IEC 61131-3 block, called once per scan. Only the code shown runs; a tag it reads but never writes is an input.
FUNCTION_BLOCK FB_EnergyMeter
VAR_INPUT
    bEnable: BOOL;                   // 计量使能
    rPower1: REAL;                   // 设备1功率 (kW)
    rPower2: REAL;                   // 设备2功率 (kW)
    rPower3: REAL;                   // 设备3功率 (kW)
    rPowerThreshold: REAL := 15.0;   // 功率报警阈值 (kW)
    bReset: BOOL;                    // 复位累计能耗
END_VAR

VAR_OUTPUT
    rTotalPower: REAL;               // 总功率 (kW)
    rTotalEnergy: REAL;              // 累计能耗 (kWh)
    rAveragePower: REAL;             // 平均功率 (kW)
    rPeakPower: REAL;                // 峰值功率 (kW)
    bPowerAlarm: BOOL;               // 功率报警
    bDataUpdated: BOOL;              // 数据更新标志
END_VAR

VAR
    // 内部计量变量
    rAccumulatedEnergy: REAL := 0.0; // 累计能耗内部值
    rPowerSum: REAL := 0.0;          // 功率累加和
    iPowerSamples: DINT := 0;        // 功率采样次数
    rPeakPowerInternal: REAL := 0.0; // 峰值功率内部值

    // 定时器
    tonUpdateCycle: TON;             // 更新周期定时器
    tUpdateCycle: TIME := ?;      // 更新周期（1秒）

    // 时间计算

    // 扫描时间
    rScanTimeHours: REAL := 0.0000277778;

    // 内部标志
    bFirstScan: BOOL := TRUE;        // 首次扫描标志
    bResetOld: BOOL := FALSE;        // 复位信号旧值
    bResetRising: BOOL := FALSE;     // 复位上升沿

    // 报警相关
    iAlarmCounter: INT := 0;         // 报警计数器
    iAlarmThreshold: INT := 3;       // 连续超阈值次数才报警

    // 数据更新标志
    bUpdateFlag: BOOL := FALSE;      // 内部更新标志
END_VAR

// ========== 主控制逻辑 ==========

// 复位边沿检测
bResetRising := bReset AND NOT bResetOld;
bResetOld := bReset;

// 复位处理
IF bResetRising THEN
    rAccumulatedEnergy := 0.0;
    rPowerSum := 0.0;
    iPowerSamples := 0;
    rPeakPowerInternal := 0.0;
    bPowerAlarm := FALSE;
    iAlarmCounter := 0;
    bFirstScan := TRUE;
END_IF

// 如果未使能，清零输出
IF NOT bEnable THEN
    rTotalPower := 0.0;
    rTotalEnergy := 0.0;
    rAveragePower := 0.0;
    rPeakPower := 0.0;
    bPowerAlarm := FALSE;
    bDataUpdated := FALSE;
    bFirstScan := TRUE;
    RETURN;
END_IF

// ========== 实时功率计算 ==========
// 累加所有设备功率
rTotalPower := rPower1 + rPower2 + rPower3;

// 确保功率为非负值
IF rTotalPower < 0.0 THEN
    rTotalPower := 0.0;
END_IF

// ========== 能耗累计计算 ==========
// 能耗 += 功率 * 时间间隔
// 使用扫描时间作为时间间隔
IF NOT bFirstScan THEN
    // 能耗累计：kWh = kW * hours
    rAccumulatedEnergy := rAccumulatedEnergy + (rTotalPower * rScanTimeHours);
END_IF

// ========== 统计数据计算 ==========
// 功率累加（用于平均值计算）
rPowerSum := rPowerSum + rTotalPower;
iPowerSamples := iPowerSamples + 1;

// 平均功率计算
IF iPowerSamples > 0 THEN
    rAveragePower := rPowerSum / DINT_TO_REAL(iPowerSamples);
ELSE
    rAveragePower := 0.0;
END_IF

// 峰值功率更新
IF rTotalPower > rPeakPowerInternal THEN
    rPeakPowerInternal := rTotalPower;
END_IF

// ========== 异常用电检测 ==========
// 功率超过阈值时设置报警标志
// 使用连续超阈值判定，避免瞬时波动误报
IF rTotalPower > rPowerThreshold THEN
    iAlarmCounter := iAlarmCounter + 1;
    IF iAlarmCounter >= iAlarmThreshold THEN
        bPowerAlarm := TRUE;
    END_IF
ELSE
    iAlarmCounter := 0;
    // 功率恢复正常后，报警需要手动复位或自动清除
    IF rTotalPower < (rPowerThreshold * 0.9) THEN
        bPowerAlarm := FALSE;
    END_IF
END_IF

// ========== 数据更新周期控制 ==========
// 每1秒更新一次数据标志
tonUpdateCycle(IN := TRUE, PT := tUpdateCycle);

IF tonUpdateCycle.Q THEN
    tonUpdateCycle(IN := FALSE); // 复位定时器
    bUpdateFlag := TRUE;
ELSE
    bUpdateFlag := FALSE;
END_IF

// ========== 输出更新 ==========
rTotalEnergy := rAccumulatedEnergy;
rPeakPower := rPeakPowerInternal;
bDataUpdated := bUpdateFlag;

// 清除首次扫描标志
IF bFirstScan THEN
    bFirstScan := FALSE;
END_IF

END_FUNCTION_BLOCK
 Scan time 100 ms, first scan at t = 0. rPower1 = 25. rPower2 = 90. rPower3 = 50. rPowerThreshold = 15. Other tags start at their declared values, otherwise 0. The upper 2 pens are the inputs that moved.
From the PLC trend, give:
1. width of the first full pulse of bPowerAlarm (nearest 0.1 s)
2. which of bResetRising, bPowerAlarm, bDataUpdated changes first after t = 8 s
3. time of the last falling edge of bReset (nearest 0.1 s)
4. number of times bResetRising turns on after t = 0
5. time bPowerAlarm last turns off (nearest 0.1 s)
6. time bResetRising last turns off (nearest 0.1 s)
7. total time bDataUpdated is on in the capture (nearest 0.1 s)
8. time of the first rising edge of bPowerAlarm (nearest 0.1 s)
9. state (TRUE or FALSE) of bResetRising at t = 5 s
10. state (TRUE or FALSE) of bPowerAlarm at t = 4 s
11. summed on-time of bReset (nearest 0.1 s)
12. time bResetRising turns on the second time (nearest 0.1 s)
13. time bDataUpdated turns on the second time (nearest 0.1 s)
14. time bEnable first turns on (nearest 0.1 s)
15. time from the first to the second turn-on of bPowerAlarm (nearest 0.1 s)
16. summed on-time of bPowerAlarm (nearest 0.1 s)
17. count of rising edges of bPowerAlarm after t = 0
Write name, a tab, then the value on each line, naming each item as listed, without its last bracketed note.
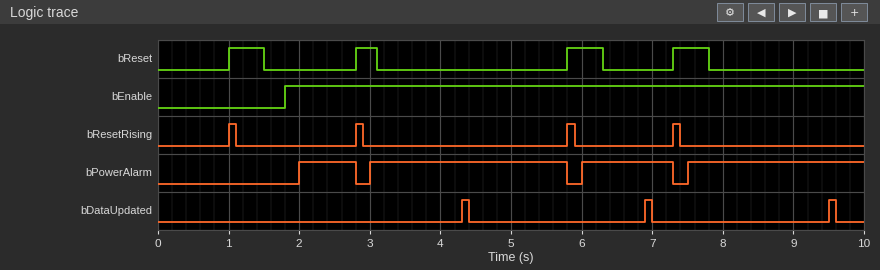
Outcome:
width of the first full pulse of bPowerAlarm	0.8 s
which of bResetRising, bPowerAlarm, bDataUpdated changes first after t = 8 s	bDataUpdated
time of the last falling edge of bReset	7.8 s
number of times bResetRising turns on after t = 0	4
time bPowerAlarm last turns off	7.3 s
time bResetRising last turns off	7.4 s
total time bDataUpdated is on in the capture	0.3 s
time of the first rising edge of bPowerAlarm	2.0 s
state (TRUE or FALSE) of bResetRising at t = 5 s	FALSE
state (TRUE or FALSE) of bPowerAlarm at t = 4 s	TRUE
summed on-time of bReset	1.8 s
time bResetRising turns on the second time	2.8 s
time bDataUpdated turns on the second time	6.9 s
time bEnable first turns on	1.8 s
time from the first to the second turn-on of bPowerAlarm	1.0 s
summed on-time of bPowerAlarm	7.4 s
count of rising edges of bPowerAlarm after t = 0	4
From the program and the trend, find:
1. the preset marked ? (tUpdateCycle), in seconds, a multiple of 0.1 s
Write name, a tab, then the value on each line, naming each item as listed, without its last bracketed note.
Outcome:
the preset marked ? (tUpdateCycle), in seconds, a multiple of 0.1 s	2.5 s
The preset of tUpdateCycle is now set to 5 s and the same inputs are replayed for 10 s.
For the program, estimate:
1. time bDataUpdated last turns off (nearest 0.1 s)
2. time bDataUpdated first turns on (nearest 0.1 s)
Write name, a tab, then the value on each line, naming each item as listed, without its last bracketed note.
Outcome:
time bDataUpdated last turns off	6.9 s
time bDataUpdated first turns on	6.8 s
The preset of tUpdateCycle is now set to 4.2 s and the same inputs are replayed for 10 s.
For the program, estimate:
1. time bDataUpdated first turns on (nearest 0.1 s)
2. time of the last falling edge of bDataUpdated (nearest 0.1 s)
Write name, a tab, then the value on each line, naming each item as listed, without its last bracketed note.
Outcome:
time bDataUpdated first turns on	6.0 s
time of the last falling edge of bDataUpdated	6.1 s
